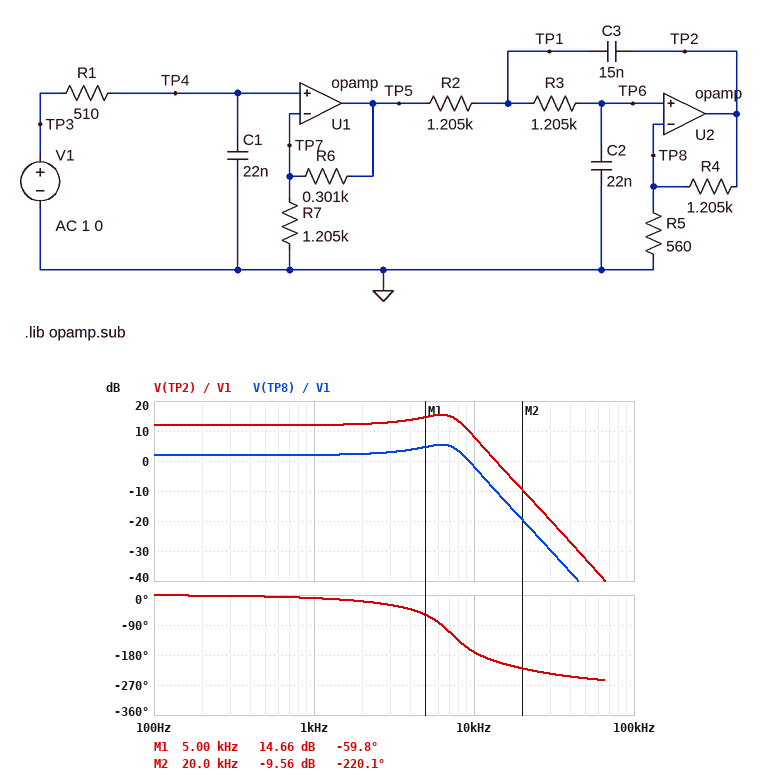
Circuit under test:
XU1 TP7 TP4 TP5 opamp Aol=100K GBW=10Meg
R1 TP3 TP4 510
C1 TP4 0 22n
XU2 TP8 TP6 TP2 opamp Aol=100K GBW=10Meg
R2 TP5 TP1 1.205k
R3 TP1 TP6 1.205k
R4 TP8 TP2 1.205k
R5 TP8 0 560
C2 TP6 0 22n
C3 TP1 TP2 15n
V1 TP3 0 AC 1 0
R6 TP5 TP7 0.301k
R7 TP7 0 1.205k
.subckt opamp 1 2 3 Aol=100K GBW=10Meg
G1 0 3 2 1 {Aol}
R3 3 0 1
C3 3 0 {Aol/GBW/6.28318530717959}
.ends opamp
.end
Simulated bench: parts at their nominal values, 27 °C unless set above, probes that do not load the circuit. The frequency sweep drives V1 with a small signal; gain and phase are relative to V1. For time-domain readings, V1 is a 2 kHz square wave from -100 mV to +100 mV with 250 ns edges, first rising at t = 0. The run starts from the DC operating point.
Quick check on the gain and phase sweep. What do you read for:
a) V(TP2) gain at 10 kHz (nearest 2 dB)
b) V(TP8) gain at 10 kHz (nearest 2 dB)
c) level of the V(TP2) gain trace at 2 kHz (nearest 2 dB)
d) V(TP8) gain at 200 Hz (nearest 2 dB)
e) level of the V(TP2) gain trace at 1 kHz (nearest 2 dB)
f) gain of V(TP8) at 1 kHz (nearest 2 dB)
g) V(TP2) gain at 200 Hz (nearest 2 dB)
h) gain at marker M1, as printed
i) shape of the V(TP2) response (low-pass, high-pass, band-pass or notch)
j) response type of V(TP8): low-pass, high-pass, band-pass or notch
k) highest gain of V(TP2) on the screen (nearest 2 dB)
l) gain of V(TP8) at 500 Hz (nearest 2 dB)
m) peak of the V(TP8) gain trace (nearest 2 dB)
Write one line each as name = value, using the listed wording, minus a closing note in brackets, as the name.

V(TP2) gain at 10 kHz = 8 dB
V(TP8) gain at 10 kHz = -2 dB
level of the V(TP2) gain trace at 2 kHz = 12 dB
V(TP8) gain at 200 Hz = 2 dB
level of the V(TP2) gain trace at 1 kHz = 12 dB
gain of V(TP8) at 1 kHz = 2 dB
V(TP2) gain at 200 Hz = 12 dB
gain at marker M1, as printed = 14.66 dB
shape of the V(TP2) response = low-pass
response type of V(TP8): low-pass, high-pass, band-pass or notch = low-pass
highest gain of V(TP2) on the screen = 16 dB
gain of V(TP8) at 500 Hz = 2 dB
peak of the V(TP8) gain trace = 6 dB
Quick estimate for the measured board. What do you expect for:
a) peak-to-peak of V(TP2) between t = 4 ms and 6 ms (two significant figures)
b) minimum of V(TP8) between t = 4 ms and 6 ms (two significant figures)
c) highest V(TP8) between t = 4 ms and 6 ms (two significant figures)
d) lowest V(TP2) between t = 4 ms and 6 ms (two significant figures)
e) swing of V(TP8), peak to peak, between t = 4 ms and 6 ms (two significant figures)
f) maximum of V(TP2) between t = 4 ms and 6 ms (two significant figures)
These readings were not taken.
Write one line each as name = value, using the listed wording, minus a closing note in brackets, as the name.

peak-to-peak of V(TP2) between t = 4 ms and 6 ms = 1.3 V
minimum of V(TP8) between t = 4 ms and 6 ms = -200 mV
highest V(TP8) between t = 4 ms and 6 ms = 200 mV
lowest V(TP2) between t = 4 ms and 6 ms = -630 mV
swing of V(TP8), peak to peak, between t = 4 ms and 6 ms = 400 mV
maximum of V(TP2) between t = 4 ms and 6 ms = 630 mV
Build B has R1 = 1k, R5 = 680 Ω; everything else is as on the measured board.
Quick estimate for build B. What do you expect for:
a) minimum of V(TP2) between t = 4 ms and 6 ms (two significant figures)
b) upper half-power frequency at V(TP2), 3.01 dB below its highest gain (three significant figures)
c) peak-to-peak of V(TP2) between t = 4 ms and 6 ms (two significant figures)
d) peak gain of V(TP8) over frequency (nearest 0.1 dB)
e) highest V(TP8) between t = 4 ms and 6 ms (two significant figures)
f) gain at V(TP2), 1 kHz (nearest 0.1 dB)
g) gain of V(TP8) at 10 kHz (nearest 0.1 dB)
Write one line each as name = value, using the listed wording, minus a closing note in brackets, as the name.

minimum of V(TP2) between t = 4 ms and 6 ms = -410 mV
upper half-power frequency at V(TP2), 3.01 dB below its highest gain = 7.43 kHz
peak-to-peak of V(TP2) between t = 4 ms and 6 ms = 820 mV
peak gain of V(TP8) over frequency = 2.0 dB
highest V(TP8) between t = 4 ms and 6 ms = 150 mV
gain at V(TP2), 1 kHz = 10.8 dB
gain of V(TP8) at 10 kHz = -6.8 dB
